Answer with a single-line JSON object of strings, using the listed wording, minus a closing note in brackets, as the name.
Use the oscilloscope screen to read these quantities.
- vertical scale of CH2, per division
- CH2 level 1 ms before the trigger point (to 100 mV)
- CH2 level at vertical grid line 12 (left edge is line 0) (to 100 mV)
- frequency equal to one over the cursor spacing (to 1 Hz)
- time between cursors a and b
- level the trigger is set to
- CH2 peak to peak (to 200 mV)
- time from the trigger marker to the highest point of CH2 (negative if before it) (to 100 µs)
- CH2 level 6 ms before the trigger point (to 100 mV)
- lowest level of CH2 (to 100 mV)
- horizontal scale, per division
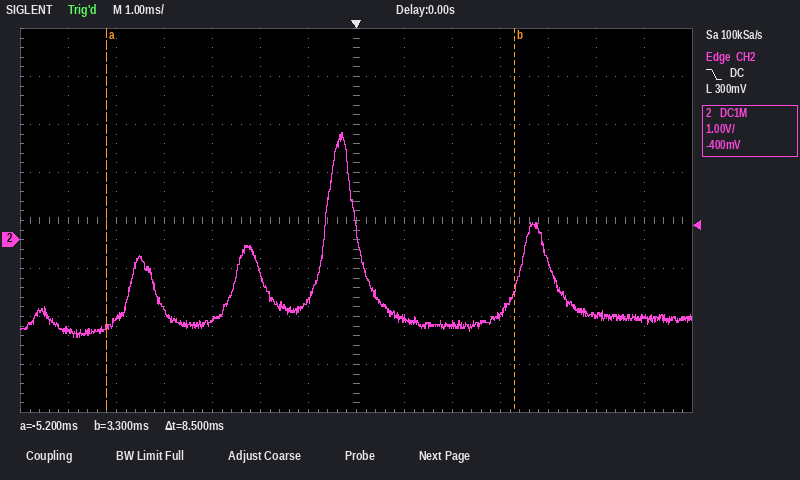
{"vertical scale of CH2, per division": "1 V", "CH2 level 1 ms before the trigger point": "-1.3 V", "CH2 level at vertical grid line 12 (left edge is line 0)": "-1.6 V", "frequency equal to one over the cursor spacing": "118 Hz", "time between cursors a and b": "8.5 ms", "level the trigger is set to": "300 mV", "CH2 peak to peak": "4.2 V", "time from the trigger marker to the highest point of CH2 (negative if before it)": "-300 µs", "CH2 level 6 ms before the trigger point": "-1.9 V", "lowest level of CH2": "-2.0 V", "horizontal scale, per division": "1 ms"}
